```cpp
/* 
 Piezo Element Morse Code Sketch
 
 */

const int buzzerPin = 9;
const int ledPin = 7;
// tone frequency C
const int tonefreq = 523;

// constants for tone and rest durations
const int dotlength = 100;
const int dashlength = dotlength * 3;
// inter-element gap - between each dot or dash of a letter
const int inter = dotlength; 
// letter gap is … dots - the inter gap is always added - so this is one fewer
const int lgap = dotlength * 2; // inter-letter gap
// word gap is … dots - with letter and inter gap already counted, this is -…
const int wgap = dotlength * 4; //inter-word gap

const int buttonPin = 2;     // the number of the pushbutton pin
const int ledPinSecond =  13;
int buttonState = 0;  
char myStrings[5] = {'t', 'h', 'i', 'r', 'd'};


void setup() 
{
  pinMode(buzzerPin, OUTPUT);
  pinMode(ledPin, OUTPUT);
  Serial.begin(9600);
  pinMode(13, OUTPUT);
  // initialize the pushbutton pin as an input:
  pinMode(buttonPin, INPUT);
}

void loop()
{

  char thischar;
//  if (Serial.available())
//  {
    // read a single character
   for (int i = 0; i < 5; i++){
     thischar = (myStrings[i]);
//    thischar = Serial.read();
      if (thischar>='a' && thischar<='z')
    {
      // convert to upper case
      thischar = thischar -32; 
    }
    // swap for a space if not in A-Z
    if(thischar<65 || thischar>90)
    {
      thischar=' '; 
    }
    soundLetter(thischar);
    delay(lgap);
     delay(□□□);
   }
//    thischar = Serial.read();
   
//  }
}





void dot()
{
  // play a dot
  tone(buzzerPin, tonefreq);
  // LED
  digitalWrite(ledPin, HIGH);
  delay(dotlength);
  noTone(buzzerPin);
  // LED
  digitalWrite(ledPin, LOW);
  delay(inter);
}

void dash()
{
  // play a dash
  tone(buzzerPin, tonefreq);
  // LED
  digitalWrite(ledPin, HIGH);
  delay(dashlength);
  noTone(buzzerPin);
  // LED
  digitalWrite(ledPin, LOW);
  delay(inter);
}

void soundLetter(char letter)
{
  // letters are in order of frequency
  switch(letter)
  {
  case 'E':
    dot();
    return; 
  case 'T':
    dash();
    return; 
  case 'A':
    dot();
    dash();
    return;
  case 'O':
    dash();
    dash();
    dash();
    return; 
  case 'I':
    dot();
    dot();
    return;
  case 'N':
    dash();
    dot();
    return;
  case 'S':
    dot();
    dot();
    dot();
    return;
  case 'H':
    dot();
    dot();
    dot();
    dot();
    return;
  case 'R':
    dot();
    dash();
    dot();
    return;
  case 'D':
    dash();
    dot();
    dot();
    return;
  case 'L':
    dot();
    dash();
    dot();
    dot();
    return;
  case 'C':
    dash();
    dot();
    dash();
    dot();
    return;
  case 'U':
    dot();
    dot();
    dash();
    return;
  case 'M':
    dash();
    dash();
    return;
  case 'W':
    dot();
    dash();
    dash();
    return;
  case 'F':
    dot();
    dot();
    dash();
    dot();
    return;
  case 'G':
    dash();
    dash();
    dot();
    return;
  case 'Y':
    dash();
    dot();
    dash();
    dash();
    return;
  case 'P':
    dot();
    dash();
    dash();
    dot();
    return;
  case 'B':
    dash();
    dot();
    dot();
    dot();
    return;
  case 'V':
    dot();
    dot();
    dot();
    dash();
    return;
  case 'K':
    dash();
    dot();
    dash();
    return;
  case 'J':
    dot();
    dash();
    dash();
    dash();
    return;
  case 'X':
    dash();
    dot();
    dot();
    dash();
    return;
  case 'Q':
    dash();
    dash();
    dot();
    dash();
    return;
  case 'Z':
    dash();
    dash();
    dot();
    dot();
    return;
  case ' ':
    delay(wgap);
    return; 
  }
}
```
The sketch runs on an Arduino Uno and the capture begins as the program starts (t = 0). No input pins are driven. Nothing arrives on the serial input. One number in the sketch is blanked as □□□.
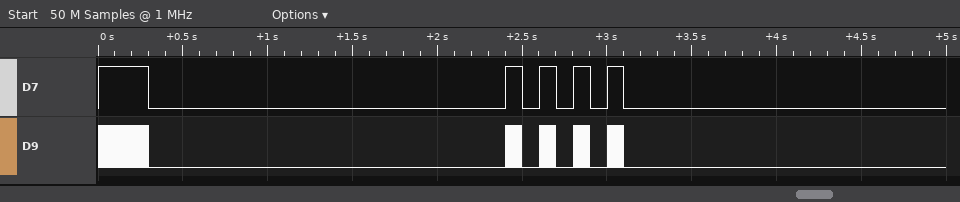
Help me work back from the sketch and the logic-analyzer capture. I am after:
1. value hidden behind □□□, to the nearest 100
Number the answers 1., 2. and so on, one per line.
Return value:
1. 1800
